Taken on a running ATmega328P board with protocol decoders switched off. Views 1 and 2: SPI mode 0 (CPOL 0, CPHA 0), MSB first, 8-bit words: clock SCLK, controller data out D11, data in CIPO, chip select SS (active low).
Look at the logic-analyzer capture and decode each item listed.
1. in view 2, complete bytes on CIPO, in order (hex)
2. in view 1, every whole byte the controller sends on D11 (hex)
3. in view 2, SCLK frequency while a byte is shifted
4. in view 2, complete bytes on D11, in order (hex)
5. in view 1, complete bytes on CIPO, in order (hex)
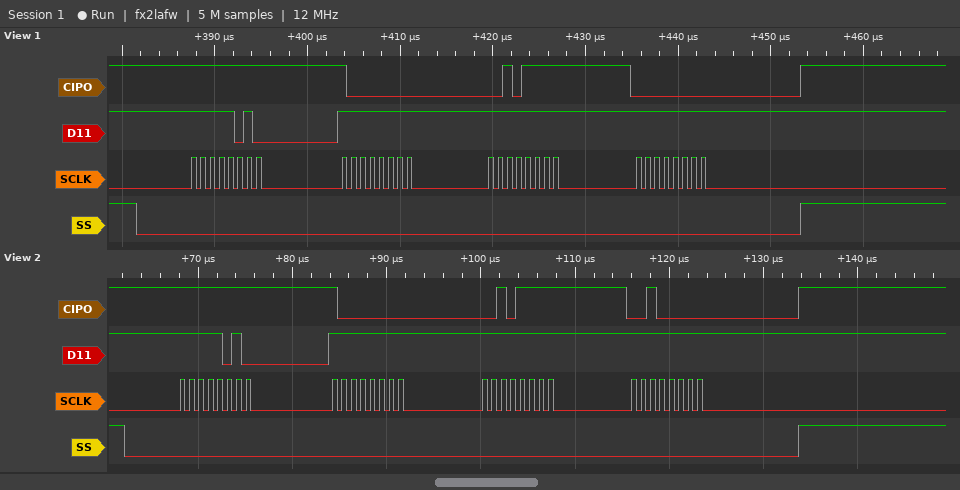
FF 80 2F 20
0xFA 0xFF 0xFF 0xFF
1 MHz
FA FF FF FF
0xFF 0x80 0x2F 0x00
